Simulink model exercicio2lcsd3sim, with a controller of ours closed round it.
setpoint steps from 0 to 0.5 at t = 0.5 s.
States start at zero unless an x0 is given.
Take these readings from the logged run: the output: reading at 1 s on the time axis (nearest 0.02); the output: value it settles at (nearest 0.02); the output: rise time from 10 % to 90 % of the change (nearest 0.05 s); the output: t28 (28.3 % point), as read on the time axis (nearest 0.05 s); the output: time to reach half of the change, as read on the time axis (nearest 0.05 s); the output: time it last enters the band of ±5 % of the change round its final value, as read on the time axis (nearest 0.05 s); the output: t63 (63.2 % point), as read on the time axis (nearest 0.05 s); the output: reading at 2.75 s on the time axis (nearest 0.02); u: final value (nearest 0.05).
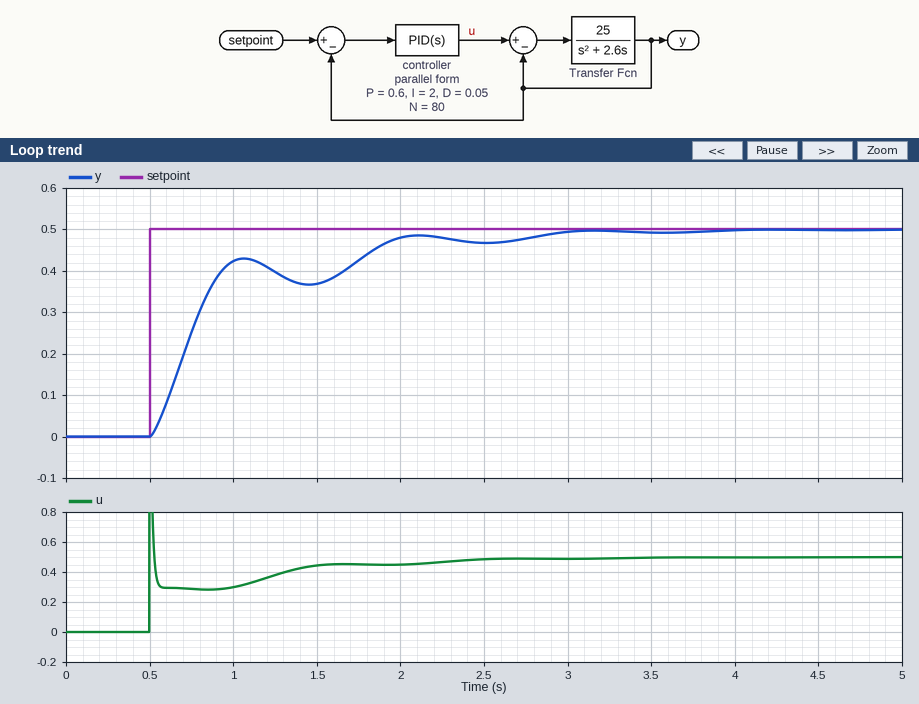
0.42
0.50
1.25 s
0.65 s
0.75 s
2.70 s
0.80 s
0.48
0.50
